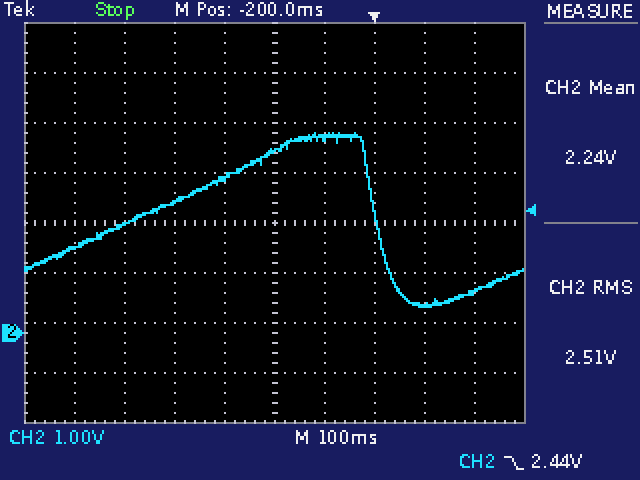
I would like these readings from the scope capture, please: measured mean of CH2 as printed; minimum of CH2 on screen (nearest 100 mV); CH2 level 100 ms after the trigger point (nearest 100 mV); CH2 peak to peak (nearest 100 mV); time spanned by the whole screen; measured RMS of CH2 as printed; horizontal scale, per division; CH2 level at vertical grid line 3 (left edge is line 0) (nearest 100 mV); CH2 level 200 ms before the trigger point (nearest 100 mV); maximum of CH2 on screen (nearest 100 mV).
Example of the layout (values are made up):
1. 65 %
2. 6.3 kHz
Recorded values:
1. 2.24 V
2. 500 mV
3. 600 mV
4. 3.5 V
5. 1 s
6. 2.51 V
7. 100 ms
8. 2.6 V
9. 3.6 V
10. 4.0 V
